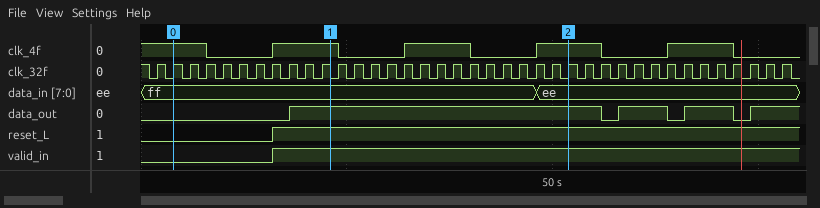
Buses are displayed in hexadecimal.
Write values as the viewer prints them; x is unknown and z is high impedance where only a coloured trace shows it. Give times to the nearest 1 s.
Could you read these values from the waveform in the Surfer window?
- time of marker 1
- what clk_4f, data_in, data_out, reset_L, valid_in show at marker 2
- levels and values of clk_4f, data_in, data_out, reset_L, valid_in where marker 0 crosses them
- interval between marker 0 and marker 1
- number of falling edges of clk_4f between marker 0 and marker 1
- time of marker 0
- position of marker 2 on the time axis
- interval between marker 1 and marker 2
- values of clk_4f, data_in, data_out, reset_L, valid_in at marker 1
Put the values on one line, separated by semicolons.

23 s; clk_4f=1, data_in=ee, data_out=1, reset_L=1, valid_in=1; clk_4f=1, data_in=ff, data_out=0, reset_L=0, valid_in=0; 19 s; 1; 4 s; 52 s; 29 s; clk_4f=1, data_in=ff, data_out=1, reset_L=1, valid_in=1
